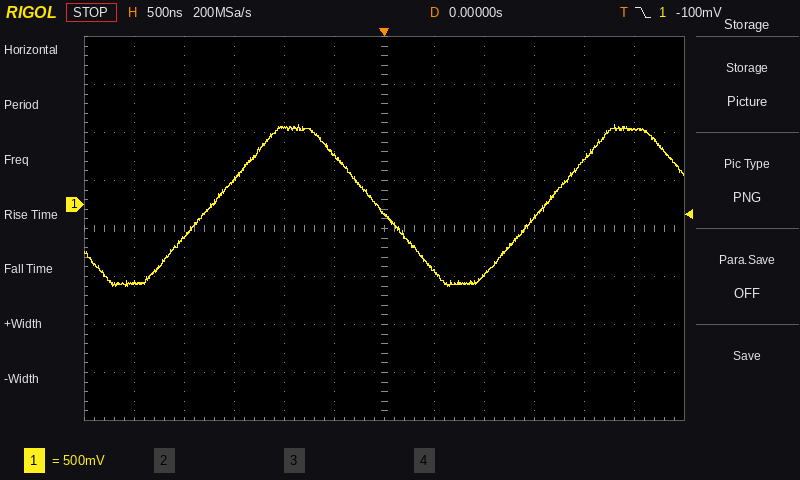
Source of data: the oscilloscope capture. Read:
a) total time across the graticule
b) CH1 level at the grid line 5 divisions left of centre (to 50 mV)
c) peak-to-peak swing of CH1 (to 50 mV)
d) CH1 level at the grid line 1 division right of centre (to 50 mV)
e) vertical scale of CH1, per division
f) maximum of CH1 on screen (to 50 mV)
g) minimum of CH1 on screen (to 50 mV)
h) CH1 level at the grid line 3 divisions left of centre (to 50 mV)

6 µs
-800 mV
1.70 V
-700 mV
500 mV
850 mV
-850 mV
250 mV
